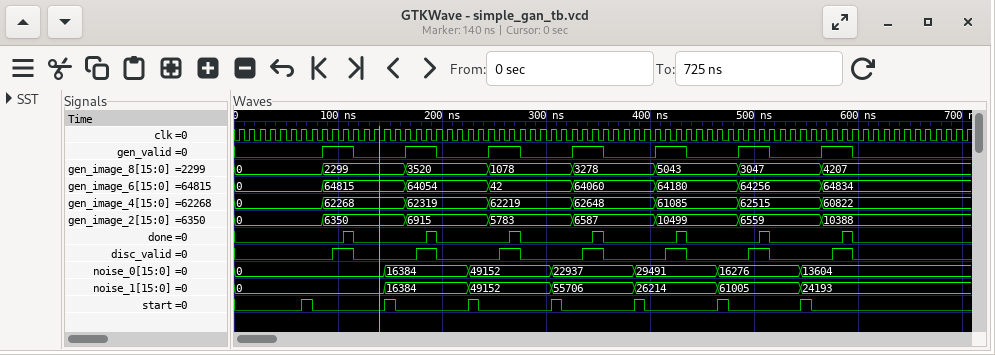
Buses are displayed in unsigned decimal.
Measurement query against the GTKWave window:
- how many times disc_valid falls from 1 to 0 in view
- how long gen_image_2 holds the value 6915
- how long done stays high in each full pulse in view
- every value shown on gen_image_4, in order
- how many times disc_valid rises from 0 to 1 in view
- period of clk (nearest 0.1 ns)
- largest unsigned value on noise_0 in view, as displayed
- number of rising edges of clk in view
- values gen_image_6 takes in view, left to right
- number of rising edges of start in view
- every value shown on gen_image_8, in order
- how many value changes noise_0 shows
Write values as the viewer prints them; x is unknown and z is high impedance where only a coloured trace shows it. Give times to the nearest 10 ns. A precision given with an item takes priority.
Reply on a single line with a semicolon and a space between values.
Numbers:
7; 80 ns; 10 ns, 10 ns, 10 ns, 10 ns, 10 ns, 10 ns, 10 ns; 0, 62268, 62319, 62219, 62648, 61085, 62515, 60822; 7; 10 ns; 49152; 71; 0, 64815, 64054, 42, 64060, 64180, 64256, 64834; 7; 0, 2299, 3520, 1078, 3278, 5043, 3047, 4207; 6
